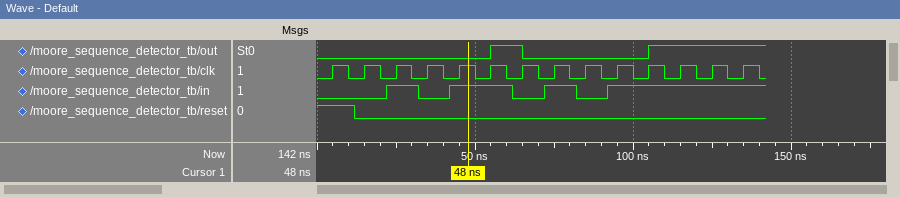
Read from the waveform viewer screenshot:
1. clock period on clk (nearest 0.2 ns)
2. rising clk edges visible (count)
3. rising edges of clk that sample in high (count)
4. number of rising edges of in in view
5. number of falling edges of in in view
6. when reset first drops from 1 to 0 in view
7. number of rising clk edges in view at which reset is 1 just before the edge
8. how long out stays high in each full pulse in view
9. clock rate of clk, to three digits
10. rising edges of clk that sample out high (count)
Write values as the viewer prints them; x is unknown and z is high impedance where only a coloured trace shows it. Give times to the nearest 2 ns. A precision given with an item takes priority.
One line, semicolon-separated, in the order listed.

10 ns; 14; 9; 4; 3; 12 ns; 1; 10 ns; 100 MHz; 4
